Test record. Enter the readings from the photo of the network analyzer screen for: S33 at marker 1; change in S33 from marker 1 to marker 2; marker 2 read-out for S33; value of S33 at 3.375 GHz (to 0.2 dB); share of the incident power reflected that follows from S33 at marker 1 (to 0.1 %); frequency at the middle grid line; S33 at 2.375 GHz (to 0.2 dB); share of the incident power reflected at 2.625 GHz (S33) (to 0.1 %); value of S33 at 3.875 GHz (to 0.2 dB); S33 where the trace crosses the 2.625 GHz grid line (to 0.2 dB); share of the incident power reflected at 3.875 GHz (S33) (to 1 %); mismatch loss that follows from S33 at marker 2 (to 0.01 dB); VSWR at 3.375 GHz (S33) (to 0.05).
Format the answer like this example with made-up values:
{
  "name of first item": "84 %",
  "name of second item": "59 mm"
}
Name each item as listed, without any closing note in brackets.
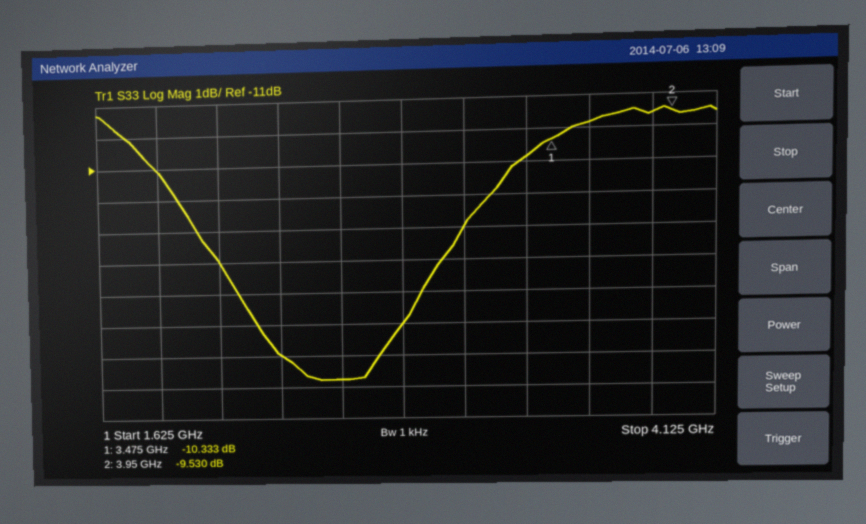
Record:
{
  "S33 at marker 1": "-10.333 dB",
  "change in S33 from marker 1 to marker 2": "0.803 dB",
  "marker 2 read-out for S33": "-9.530 dB",
  "value of S33 at 3.375 GHz": "-10.8 dB",
  "share of the incident power reflected that follows from S33 at marker 1": "9.3 %",
  "frequency at the middle grid line": "2.875 GHz",
  "S33 at 2.375 GHz": "-17.0 dB",
  "share of the incident power reflected at 2.625 GHz (S33)": "1.7 %",
  "value of S33 at 3.875 GHz": "-9.6 dB",
  "S33 where the trace crosses the 2.625 GHz grid line": "-17.8 dB",
  "share of the incident power reflected at 3.875 GHz (S33)": "11 %",
  "mismatch loss that follows from S33 at marker 2": "0.51 dB",
  "VSWR at 3.375 GHz (S33)": "1.80"
}
